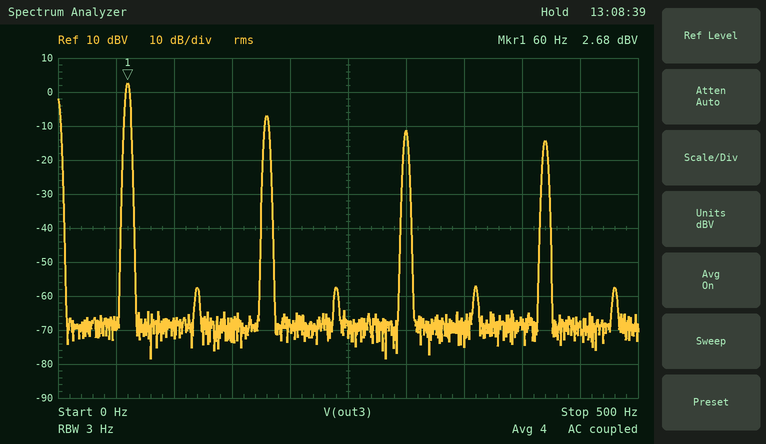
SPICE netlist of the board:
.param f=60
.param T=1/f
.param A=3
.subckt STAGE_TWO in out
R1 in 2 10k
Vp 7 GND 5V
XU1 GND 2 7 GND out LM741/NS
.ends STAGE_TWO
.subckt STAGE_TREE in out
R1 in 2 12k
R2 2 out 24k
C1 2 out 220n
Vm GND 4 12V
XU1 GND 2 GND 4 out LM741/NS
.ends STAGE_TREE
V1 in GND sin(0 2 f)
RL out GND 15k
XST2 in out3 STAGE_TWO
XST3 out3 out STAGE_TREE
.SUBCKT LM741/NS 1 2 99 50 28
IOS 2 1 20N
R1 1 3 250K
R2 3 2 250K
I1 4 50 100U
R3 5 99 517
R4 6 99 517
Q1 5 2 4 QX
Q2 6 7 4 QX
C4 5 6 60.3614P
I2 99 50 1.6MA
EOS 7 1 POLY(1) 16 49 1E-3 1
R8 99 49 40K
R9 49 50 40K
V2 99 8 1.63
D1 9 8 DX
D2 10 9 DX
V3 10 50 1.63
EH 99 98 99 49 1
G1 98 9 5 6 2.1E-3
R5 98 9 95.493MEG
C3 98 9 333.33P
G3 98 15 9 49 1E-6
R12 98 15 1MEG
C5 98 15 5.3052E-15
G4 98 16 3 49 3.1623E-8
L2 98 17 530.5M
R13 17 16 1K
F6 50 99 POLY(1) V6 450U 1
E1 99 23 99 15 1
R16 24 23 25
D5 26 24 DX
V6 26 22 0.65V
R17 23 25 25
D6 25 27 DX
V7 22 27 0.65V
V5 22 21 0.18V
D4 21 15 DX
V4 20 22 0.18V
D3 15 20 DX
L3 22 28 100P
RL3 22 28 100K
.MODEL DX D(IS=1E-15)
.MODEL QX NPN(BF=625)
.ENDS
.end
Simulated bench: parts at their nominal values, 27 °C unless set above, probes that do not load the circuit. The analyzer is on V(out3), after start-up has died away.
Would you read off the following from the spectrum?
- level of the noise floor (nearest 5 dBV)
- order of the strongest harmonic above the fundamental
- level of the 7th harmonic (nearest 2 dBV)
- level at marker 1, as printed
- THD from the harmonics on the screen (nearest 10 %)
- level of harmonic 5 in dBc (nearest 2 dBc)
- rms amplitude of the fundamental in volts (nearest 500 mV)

-70 dBV
3
-14 dBV
2.68 dBV
40 %
-14 dBc
1.5 V
